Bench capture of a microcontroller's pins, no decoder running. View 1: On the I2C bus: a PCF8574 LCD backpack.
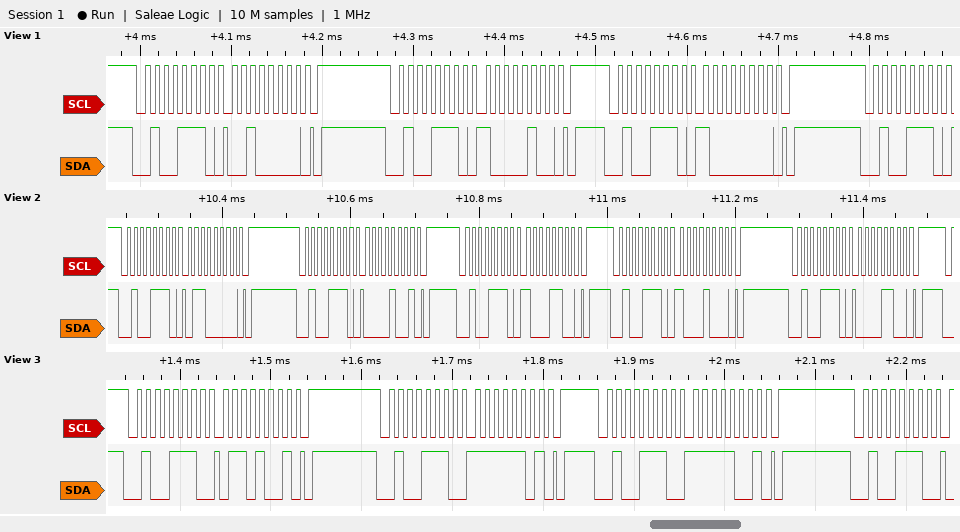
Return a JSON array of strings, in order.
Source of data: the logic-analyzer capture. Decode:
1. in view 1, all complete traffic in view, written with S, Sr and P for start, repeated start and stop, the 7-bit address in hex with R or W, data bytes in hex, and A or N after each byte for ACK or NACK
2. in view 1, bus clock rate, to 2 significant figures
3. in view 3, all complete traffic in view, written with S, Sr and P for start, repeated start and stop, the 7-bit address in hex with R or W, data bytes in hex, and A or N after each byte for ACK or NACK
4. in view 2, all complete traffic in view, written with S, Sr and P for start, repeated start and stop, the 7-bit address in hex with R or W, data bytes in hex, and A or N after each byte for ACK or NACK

["S 27W A 20 A P S 27W A 84 A P S 27W A 80 A P S 27W A", "100 kHz", "S 27W A 69 A P S 27W A FD A P S 27W A F9 A P S 27W A", "S 27W A 60 A P S 27W A 09 A P S 27W A 8C A P S 27W A 88 A P S 27W A 0C A P"]
